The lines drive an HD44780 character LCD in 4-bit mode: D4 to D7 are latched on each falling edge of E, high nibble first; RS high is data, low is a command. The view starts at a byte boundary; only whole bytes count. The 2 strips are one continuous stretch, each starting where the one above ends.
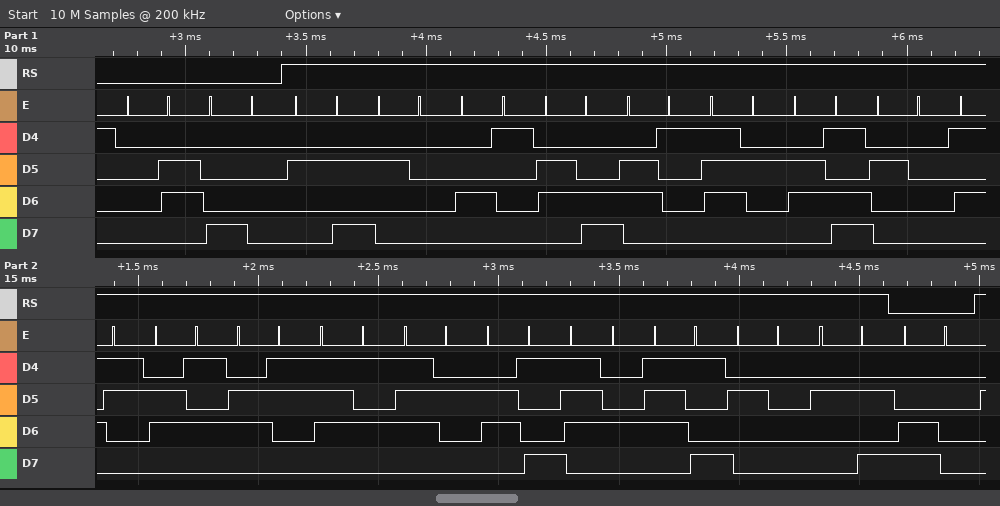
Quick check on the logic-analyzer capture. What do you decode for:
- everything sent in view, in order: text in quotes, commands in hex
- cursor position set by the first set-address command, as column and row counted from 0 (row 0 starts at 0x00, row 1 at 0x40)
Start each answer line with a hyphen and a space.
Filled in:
- 0x06 0x80 "* Alarm Security *" 0xC0
- column 0, row 0
